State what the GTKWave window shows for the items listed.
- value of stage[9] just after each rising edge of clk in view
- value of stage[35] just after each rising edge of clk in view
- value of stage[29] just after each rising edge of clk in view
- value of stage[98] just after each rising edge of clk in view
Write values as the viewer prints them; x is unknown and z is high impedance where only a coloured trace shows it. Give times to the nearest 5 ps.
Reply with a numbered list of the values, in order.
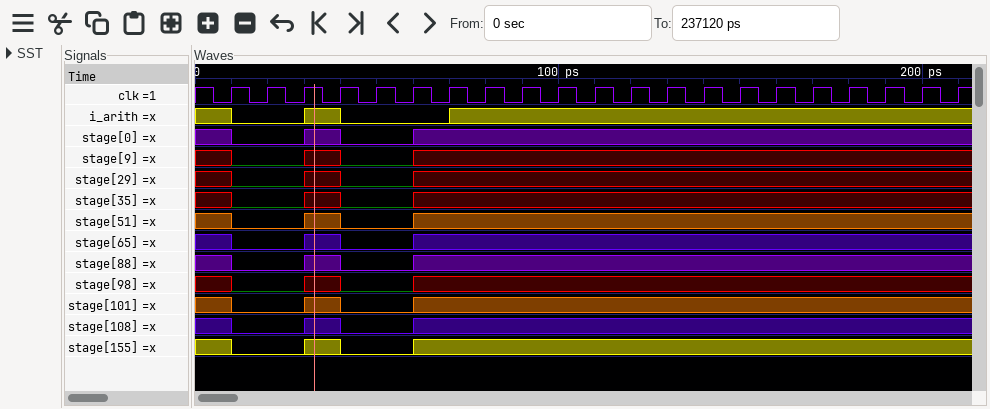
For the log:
1. 0 0 x 0 0 x x x x x x x x x x x x x x x x
2. 0 0 x 0 0 x x x x x x x x x x x x x x x x
3. 0 0 x 0 0 x x x x x x x x x x x x x x x x
4. 0 0 x 0 0 x x x x x x x x x x x x x x x x
